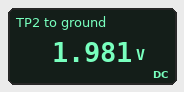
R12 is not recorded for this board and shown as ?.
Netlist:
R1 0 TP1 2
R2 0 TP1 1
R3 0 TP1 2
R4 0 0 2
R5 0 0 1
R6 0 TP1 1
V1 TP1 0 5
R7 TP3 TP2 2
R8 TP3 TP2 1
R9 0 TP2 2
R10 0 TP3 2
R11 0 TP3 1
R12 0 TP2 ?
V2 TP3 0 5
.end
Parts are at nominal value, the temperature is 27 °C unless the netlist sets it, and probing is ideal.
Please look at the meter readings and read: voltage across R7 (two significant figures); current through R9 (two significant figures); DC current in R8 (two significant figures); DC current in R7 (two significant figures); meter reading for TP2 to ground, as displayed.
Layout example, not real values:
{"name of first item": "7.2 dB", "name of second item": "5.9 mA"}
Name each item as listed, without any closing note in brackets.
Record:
{"voltage across R7": "3.0 V", "current through R9": "990 mA", "DC current in R8": "3.0 A", "DC current in R7": "1.5 A", "meter reading for TP2 to ground, as displayed": "1.981 V"}
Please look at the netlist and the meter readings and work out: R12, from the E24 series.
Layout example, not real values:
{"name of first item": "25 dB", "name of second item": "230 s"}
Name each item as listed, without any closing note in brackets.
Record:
{"R12, from the E24 series": "0.56 Ω"}
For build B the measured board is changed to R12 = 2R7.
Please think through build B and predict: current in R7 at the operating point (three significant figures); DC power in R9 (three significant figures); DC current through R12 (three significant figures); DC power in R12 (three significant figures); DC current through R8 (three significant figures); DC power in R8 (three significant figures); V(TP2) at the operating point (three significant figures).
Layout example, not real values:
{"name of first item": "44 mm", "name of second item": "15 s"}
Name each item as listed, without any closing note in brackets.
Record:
{"current in R7 at the operating point": "918 mA", "DC power in R9": "5.01 W", "DC current through R12": "1.17 A", "DC power in R12": "3.71 W", "DC current through R8": "1.84 A", "DC power in R8": "3.37 W", "V(TP2) at the operating point": "3.16 V"}
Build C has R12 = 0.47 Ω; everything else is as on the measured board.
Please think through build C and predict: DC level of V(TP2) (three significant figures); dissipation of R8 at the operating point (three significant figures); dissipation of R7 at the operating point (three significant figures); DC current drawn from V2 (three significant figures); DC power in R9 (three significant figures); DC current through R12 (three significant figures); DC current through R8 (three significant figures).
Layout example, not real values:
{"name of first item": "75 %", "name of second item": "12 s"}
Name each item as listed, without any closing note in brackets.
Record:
{"DC level of V(TP2)": "1.82 V", "dissipation of R8 at the operating point": "10.1 W", "dissipation of R7 at the operating point": "5.07 W", "DC current drawn from V2": "12.3 A", "DC power in R9": "1.65 W", "DC current through R12": "3.87 A", "DC current through R8": "3.18 A"}
